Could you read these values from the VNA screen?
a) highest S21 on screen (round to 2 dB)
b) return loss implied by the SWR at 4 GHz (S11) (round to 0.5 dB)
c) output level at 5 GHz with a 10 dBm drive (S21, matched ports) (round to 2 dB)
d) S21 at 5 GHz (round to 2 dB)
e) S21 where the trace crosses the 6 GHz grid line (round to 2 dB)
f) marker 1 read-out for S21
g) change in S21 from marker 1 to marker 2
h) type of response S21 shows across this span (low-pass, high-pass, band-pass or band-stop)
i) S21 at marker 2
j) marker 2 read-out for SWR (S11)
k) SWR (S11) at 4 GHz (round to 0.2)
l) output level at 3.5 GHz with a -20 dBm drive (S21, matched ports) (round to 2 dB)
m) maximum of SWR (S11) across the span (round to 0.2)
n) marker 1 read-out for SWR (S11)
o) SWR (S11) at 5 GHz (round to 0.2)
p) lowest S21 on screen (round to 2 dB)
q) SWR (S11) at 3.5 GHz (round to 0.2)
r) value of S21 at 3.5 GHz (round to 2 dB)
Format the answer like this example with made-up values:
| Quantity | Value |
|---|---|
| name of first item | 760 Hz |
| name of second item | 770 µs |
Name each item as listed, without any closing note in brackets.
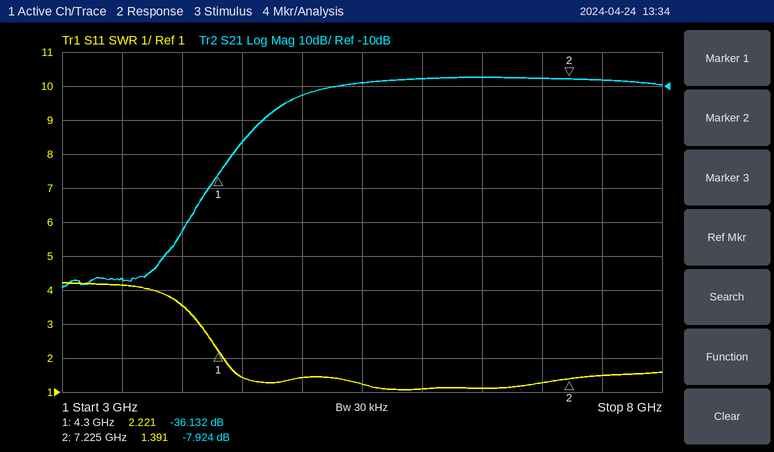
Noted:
| Quantity | Value |
|---|---|
| highest S21 on screen | -8 dB |
| return loss implied by the SWR at 4 GHz (S11) | 5.0 dB |
| output level at 5 GHz with a 10 dBm drive (S21, matched ports) | -2 dBm |
| S21 at 5 GHz | -12 dB |
| S21 where the trace crosses the 6 GHz grid line | -8 dB |
| marker 1 read-out for S21 | -36.132 dB |
| change in S21 from marker 1 to marker 2 | 28.208 dB |
| type of response S21 shows across this span | high-pass |
| S21 at marker 2 | -7.924 dB |
| marker 2 read-out for SWR | 1.391 |
| SWR (S11) at 4 GHz | 3.6 |
| output level at 3.5 GHz with a -20 dBm drive (S21, matched ports) | -86 dBm |
| maximum of SWR (S11) across the span | 4.2 |
| marker 1 read-out for SWR | 2.221 |
| SWR (S11) at 5 GHz | 1.4 |
| lowest S21 on screen | -70 dB |
| SWR (S11) at 3.5 GHz | 4.2 |
| value of S21 at 3.5 GHz | -66 dB |
